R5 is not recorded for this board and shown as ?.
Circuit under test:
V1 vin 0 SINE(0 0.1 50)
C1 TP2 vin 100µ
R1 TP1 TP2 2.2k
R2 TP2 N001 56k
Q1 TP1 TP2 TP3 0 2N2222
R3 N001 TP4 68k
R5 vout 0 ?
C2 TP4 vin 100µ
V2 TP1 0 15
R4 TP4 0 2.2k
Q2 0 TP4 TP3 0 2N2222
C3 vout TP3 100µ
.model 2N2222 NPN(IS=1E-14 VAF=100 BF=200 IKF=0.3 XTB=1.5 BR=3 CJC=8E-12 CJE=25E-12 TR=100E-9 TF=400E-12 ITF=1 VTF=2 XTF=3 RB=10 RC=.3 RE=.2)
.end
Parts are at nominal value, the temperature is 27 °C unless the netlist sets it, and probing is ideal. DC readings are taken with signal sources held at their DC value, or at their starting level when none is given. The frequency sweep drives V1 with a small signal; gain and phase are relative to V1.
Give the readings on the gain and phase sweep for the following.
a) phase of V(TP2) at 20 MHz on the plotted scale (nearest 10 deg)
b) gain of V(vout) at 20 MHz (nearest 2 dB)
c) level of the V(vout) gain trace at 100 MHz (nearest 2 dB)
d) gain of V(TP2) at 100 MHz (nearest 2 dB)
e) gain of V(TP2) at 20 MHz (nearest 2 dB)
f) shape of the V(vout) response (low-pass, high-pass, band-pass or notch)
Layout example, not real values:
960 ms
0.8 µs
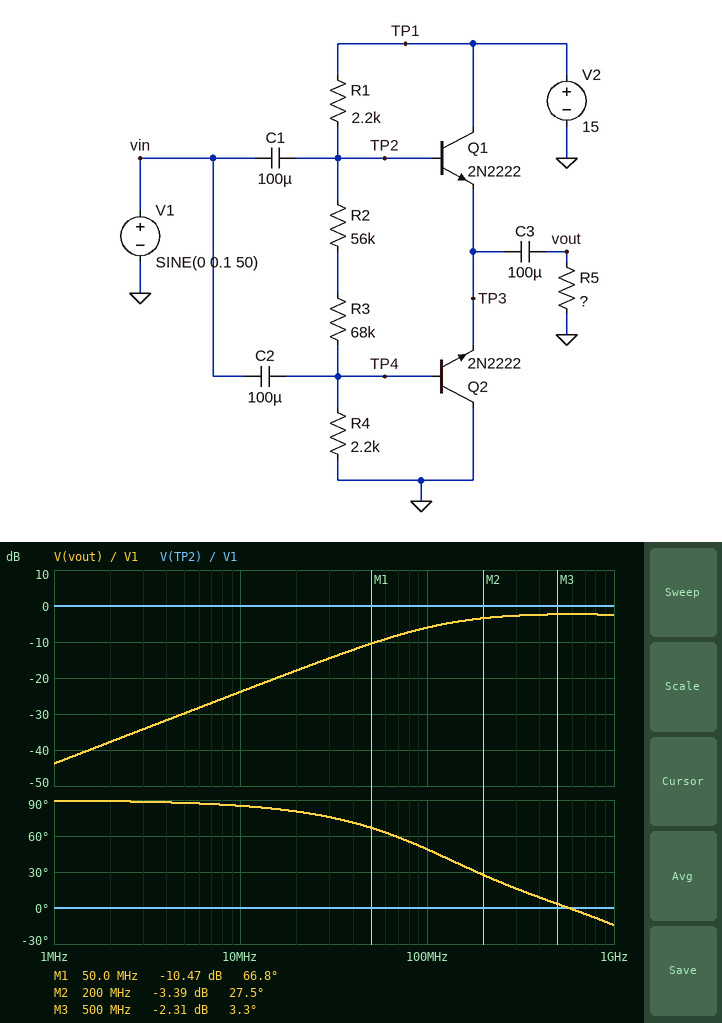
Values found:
0 deg
-18 dB
-6 dB
0 dB
0 dB
high-pass
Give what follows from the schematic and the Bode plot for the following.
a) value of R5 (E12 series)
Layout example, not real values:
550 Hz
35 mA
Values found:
27 Ω
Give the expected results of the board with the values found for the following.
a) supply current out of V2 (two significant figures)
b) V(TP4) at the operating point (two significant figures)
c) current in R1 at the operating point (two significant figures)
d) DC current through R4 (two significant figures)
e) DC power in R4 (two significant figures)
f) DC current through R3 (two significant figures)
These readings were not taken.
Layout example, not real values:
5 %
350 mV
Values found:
120 µA
260 mV
120 µA
120 µA
30 µW
120 µA
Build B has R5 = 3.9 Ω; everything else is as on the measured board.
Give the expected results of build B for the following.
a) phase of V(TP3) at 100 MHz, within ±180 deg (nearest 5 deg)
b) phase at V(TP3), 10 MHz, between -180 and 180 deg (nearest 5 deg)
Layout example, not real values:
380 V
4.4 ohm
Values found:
75 deg
90 deg
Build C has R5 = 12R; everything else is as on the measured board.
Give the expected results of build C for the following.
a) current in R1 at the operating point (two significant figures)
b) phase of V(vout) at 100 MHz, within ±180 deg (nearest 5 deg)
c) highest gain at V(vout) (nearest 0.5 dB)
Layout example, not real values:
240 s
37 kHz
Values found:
120 µA
65 deg
-4.5 dB
